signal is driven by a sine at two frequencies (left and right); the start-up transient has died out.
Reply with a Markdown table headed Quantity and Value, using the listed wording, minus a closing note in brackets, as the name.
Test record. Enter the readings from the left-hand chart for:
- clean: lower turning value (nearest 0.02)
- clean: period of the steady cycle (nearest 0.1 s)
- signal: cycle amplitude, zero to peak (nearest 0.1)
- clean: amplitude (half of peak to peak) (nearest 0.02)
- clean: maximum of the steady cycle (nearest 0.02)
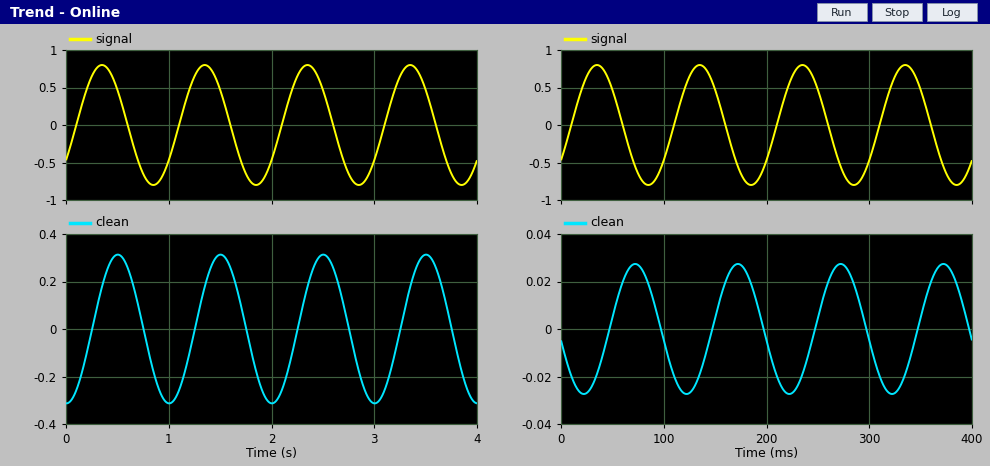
| Quantity | Value |
|---|---|
| clean: lower turning value | -0.32 |
| clean: period of the steady cycle | 1.0 s |
| signal: cycle amplitude, zero to peak | 0.8 |
| clean: amplitude (half of peak to peak) | 0.32 |
| clean: maximum of the steady cycle | 0.32 |
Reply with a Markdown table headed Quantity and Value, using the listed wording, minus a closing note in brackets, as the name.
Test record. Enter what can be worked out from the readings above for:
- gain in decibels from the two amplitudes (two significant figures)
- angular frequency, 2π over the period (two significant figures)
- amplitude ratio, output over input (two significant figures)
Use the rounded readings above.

| Quantity | Value |
|---|---|
| gain in decibels from the two amplitudes | -8.0 dB |
| angular frequency, 2π over the period | 6.3 rad/s |
| amplitude ratio, output over input | 0.40 |
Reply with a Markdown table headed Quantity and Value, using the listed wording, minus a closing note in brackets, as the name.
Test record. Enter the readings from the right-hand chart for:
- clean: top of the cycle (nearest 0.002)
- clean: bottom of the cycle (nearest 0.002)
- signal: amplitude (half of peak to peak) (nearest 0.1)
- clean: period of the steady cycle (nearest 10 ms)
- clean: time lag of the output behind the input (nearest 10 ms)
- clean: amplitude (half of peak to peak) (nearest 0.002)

| Quantity | Value |
|---|---|
| clean: top of the cycle | 0.028 |
| clean: bottom of the cycle | -0.028 |
| signal: amplitude (half of peak to peak) | 0.8 |
| clean: period of the steady cycle | 100 ms |
| clean: time lag of the output behind the input | 40 ms |
| clean: amplitude (half of peak to peak) | 0.028 |
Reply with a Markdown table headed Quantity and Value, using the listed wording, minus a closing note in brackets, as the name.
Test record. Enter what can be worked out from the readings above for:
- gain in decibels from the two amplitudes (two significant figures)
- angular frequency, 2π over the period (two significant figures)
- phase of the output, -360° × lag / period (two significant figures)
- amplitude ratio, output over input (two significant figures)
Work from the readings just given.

| Quantity | Value |
|---|---|
| gain in decibels from the two amplitudes | -29 dB |
| angular frequency, 2π over the period | 0.063 rad/ms |
| phase of the output, -360° × lag / period | -140° |
| amplitude ratio, output over input | 0.035 |
